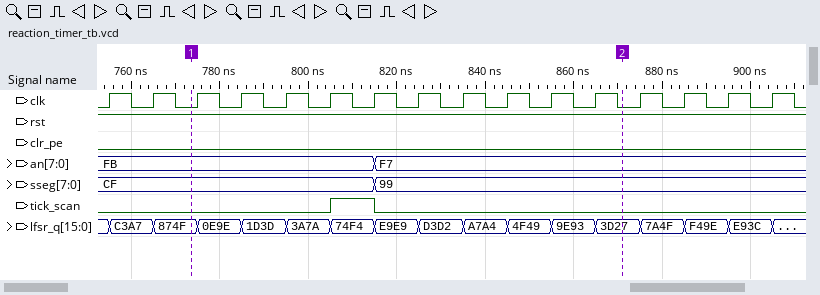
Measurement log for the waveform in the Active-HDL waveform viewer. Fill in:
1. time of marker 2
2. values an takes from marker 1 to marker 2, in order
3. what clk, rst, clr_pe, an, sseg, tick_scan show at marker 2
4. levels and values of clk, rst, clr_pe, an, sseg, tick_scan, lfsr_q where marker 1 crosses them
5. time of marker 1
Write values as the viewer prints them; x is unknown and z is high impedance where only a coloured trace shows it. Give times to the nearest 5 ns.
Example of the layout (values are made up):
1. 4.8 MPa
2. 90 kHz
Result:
1. 870 ns
2. FB, F7
3. clk=0, rst=1, clr_pe=0, an=F7, sseg=99, tick_scan=0
4. clk=0, rst=1, clr_pe=0, an=FB, sseg=CF, tick_scan=0, lfsr_q=874F
5. 775 ns
